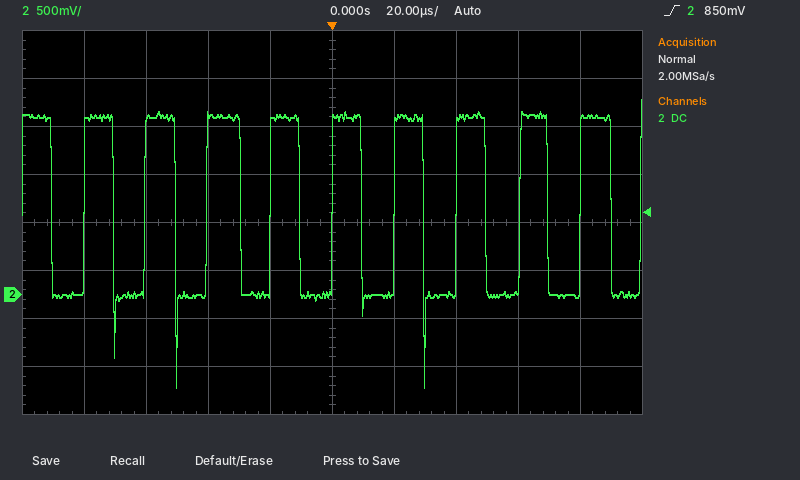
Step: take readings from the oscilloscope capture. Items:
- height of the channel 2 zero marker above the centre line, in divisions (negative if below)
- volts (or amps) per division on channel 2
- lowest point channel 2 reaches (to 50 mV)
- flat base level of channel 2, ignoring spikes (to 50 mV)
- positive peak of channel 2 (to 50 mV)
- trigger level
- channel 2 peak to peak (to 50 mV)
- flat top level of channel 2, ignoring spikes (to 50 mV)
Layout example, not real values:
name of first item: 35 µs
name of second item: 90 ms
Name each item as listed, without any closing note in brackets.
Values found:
height of the channel 2 zero marker above the centre line, in divisions: -1.5 div
volts (or amps) per division on channel 2: 500 mV
lowest point channel 2 reaches: -950 mV
flat base level of channel 2, ignoring spikes: 0 mV
positive peak of channel 2: 2.05 V
trigger level: 850 mV
channel 2 peak to peak: 3.00 V
flat top level of channel 2, ignoring spikes: 1.85 V
